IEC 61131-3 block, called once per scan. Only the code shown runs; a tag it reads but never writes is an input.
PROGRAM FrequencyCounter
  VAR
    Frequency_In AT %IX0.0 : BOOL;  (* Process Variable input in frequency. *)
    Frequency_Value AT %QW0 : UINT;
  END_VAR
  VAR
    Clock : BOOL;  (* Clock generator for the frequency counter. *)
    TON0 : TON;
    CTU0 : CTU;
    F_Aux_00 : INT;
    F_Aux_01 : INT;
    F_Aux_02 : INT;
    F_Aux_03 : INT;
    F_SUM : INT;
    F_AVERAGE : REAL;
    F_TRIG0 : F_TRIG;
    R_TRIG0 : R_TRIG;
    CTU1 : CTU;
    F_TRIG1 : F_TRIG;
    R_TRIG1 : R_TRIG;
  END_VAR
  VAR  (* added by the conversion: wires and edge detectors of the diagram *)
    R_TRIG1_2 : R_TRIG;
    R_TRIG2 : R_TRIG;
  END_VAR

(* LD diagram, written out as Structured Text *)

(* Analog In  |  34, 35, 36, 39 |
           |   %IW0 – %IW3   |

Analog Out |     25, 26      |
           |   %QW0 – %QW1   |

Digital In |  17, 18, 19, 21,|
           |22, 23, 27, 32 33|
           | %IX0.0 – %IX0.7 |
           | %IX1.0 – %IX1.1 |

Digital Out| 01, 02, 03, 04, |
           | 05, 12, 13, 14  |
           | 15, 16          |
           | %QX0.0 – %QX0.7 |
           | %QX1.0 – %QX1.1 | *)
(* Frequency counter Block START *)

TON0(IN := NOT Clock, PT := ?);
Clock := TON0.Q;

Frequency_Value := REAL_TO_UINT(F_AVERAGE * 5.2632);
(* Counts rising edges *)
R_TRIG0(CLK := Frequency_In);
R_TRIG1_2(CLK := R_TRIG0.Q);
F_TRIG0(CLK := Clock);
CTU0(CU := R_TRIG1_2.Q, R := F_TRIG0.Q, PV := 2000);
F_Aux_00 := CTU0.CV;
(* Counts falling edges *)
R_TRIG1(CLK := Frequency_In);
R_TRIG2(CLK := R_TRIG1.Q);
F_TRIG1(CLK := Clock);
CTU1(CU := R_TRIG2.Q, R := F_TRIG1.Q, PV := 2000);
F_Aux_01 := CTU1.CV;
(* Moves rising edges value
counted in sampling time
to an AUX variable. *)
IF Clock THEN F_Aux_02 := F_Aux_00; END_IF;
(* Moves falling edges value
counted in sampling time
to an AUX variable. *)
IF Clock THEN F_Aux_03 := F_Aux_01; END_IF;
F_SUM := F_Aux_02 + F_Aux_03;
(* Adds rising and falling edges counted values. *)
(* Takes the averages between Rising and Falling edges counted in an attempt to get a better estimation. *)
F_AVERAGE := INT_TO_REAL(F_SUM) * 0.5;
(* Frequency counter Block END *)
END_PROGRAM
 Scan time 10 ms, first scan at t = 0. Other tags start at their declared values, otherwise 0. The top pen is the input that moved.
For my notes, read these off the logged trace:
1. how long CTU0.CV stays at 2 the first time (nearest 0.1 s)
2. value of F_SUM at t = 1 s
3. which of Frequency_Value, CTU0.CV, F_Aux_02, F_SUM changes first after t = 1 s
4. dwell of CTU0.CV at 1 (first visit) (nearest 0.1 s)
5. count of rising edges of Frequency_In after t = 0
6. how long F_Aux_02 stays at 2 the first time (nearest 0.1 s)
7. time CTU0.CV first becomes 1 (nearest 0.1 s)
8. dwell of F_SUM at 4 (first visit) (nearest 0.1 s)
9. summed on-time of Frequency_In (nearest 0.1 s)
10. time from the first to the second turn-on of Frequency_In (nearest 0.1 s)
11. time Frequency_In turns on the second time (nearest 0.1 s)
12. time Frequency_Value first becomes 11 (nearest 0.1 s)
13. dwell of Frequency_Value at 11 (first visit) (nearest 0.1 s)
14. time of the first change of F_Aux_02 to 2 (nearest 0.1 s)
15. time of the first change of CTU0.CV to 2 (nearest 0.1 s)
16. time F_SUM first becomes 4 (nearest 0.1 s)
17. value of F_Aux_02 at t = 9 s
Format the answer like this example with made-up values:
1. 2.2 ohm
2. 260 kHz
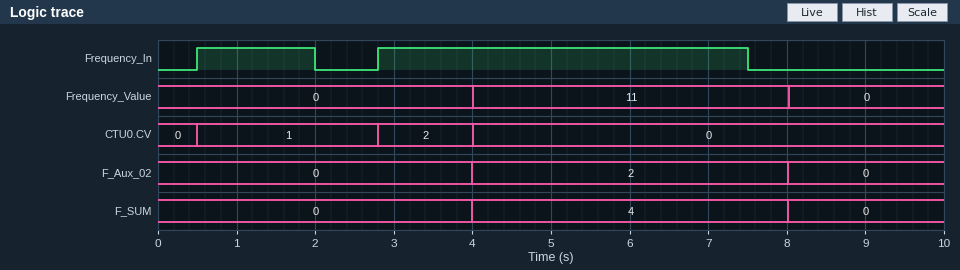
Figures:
1. 1.2 s
2. 0
3. CTU0.CV
4. 2.3 s
5. 2
6. 4.0 s
7. 0.5 s
8. 4.0 s
9. 6.2 s
10. 2.3 s
11. 2.8 s
12. 4.0 s
13. 4.0 s
14. 4.0 s
15. 2.8 s
16. 4.0 s
17. 0
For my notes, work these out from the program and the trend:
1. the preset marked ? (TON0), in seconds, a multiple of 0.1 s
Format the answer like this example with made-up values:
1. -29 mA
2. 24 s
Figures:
1. 4.0 s
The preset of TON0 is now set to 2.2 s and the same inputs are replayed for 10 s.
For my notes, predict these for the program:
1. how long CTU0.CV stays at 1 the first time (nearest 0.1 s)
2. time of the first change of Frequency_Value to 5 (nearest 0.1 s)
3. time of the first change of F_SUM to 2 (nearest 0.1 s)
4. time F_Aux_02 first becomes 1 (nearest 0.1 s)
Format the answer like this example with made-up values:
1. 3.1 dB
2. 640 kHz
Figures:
1. 1.7 s
2. 2.2 s
3. 2.2 s
4. 2.2 s
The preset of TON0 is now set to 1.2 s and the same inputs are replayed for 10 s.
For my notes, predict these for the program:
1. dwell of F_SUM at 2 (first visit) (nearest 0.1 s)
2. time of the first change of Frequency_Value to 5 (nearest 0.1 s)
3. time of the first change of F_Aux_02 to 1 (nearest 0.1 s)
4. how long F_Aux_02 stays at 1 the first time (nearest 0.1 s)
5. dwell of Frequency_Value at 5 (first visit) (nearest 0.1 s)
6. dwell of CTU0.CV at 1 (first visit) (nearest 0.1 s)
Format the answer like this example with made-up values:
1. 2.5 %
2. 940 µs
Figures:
1. 1.2 s
2. 1.2 s
3. 1.2 s
4. 1.2 s
5. 1.2 s
6. 0.7 s
